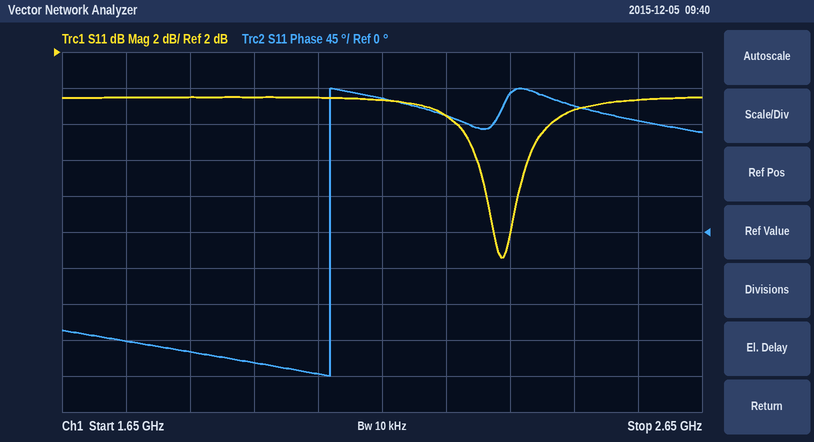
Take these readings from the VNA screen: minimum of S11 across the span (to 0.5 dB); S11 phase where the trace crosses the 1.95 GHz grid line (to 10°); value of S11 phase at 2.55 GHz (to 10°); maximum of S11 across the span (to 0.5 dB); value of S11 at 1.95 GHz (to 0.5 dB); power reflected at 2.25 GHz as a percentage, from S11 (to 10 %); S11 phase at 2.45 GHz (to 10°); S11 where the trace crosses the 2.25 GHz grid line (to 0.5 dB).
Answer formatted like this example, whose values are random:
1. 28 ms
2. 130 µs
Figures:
1. -9.5 dB
2. -160°
3. 140°
4. -0.5 dB
5. -0.5 dB
6. 70 %
7. 160°
8. -1.5 dB
